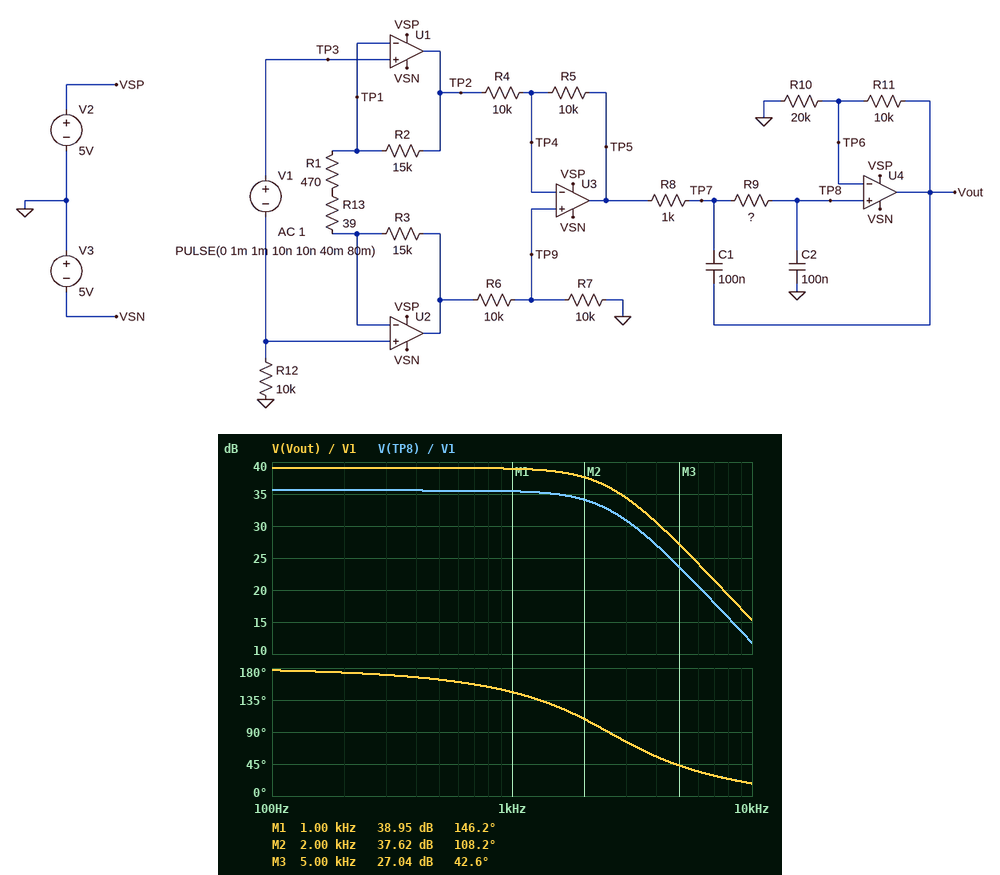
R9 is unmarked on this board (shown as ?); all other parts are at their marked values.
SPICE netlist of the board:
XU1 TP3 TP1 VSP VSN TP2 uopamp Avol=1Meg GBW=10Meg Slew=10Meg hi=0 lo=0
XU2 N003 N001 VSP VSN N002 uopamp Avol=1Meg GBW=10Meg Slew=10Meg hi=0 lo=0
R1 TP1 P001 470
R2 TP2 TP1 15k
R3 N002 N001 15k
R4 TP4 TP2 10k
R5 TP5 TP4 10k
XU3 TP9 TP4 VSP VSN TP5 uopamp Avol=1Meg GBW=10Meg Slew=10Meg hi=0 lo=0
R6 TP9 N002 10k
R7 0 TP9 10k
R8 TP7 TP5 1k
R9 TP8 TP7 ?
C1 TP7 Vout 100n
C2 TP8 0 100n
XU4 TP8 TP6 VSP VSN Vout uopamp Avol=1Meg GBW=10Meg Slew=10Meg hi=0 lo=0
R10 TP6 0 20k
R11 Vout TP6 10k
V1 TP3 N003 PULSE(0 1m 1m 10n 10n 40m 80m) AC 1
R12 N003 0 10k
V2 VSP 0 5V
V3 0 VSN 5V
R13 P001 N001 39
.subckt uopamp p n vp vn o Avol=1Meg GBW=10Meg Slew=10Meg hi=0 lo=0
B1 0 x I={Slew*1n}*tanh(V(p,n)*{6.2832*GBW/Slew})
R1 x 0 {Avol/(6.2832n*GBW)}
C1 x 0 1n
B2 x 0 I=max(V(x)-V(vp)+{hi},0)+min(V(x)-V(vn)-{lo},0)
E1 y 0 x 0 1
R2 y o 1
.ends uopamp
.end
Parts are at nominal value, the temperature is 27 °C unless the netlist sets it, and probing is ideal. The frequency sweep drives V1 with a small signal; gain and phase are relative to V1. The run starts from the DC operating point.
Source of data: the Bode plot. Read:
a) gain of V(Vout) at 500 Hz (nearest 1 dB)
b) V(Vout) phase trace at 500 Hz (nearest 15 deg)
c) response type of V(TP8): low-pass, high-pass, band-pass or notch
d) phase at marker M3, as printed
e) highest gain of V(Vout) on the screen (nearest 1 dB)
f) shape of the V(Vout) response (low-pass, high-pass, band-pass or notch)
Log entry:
39 dB
165 deg
low-pass
42.6 deg
39 dB
low-pass
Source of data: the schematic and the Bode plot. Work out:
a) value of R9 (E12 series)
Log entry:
390 Ω
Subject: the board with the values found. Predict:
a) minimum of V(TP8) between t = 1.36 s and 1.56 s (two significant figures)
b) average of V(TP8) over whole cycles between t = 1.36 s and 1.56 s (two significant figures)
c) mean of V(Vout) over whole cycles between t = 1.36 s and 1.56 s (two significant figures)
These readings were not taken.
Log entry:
-63 mV
-30 mV
-45 mV
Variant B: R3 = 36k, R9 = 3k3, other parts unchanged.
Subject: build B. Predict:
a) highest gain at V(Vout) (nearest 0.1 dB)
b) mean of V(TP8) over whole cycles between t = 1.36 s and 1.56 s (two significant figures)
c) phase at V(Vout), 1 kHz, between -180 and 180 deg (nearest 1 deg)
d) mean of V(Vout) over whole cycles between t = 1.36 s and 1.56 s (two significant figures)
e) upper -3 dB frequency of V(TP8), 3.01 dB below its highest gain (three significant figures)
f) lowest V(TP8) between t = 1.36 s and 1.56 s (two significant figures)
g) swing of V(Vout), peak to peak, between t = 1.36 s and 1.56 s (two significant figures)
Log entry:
43.6 dB
-51 mV
82 deg
-76 mV
529 Hz
-100 mV
150 mV
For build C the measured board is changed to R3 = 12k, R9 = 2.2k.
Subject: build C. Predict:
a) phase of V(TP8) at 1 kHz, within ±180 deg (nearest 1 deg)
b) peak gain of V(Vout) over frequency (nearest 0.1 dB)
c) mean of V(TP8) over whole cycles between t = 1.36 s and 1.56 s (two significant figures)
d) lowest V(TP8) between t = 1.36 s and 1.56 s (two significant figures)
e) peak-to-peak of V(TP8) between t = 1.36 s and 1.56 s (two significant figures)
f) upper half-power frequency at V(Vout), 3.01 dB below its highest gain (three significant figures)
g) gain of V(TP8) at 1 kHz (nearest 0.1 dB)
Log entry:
94 deg
38.2 dB
-27 mV
-54 mV
54 mV
788 Hz
30.0 dB
